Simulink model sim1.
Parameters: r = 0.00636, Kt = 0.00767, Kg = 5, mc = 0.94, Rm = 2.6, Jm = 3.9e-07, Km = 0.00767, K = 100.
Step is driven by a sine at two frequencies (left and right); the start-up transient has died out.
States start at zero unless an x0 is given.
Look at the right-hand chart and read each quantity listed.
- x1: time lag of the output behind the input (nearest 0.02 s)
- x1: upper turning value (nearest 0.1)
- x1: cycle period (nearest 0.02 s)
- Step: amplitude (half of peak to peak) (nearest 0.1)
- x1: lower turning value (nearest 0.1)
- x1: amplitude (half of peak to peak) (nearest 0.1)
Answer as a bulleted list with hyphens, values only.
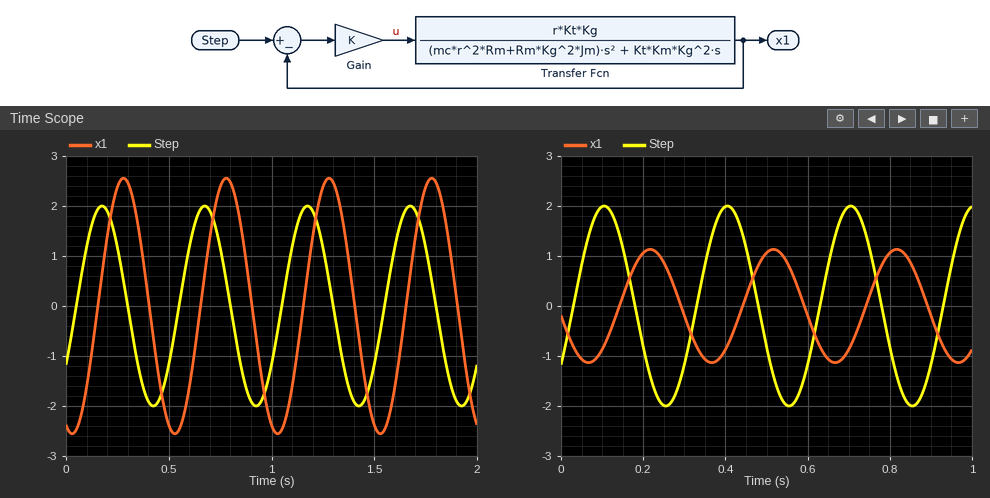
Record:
- 0.12 s
- 1.1
- 0.30 s
- 2.0
- -1.1
- 1.1
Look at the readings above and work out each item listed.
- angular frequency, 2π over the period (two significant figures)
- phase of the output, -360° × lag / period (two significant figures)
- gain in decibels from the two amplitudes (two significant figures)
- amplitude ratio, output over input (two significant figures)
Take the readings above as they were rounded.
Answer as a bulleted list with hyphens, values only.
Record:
- 21 rad/s
- -140°
- -5.2 dB
- 0.55
